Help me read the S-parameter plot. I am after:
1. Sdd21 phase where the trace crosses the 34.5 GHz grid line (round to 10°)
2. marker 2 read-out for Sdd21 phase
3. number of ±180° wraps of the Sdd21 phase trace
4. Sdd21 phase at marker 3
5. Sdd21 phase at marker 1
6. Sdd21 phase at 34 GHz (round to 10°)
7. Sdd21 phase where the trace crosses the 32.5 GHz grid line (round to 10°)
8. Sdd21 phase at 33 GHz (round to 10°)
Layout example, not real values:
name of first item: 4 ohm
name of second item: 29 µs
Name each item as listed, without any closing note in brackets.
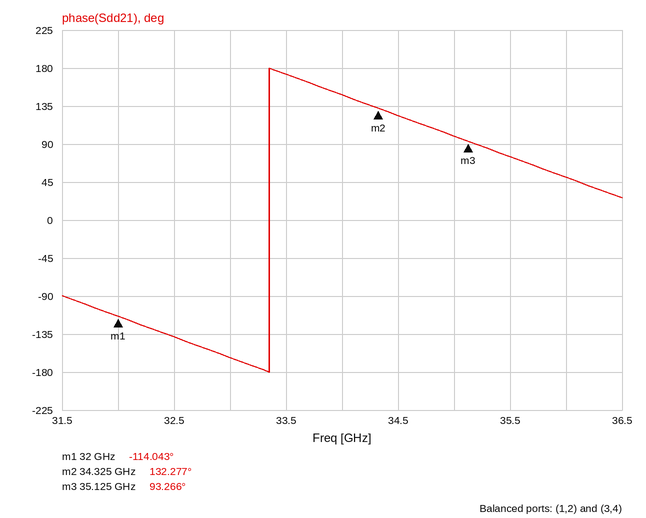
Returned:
Sdd21 phase where the trace crosses the 34.5 GHz grid line: 120°
marker 2 read-out for Sdd21 phase: 132.277°
number of ±180° wraps of the Sdd21 phase trace: 1
Sdd21 phase at marker 3: 93.266°
Sdd21 phase at marker 1: -114.043°
Sdd21 phase at 34 GHz: 150°
Sdd21 phase where the trace crosses the 32.5 GHz grid line: -140°
Sdd21 phase at 33 GHz: -160°
